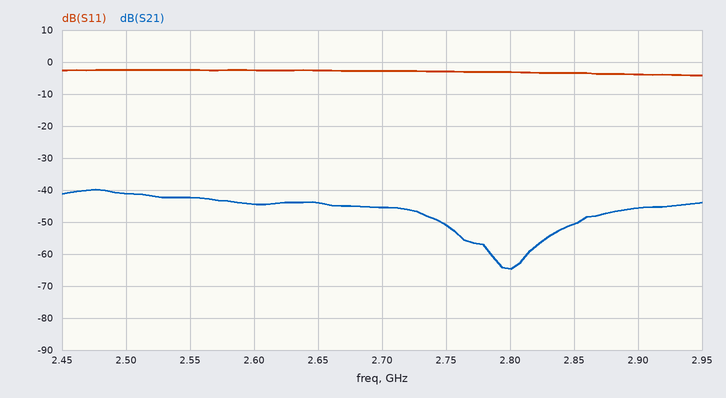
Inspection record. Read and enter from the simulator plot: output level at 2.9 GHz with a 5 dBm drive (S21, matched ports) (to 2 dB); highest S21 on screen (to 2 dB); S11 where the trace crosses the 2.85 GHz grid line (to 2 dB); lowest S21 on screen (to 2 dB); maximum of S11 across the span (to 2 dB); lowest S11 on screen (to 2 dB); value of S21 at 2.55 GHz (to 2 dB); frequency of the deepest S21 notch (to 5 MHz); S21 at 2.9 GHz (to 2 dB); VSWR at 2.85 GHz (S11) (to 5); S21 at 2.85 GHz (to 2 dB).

-40 dBm
-40 dB
-4 dB
-64 dB
-2 dB
-4 dB
-42 dB
2.800 GHz
-46 dB
5
-50 dB
